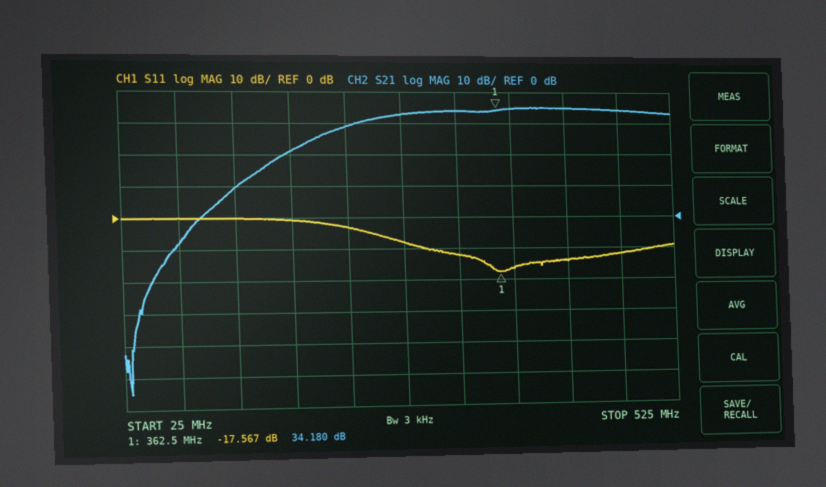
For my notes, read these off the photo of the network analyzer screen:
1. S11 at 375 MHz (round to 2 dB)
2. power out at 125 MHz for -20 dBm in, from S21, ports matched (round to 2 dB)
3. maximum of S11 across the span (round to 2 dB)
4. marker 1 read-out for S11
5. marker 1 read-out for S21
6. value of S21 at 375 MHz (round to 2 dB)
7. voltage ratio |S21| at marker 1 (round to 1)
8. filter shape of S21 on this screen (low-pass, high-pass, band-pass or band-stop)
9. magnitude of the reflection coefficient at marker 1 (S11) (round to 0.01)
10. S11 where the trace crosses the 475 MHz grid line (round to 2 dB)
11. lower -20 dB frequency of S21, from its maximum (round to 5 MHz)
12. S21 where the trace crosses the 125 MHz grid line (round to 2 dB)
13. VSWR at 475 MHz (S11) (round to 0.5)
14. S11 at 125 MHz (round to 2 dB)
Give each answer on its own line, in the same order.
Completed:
-16 dB
-10 dBm
0 dB
-17.567 dB
34.180 dB
34 dB
51
high-pass
0.13
-12 dB
150 MHz
10 dB
1.5
0 dB
